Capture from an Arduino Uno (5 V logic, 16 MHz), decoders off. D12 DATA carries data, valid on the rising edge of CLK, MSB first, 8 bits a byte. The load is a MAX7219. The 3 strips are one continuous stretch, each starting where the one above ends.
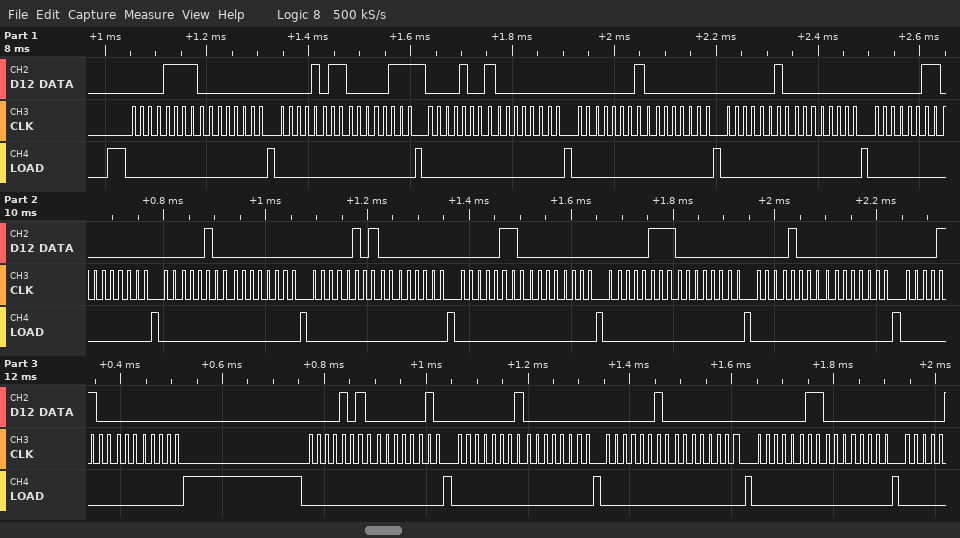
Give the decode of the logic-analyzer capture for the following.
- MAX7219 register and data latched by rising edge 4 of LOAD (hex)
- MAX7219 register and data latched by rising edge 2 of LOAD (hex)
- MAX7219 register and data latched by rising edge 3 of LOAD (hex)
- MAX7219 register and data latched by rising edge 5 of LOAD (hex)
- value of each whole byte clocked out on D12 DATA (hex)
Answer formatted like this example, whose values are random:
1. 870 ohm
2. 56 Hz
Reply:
1. register 0x9, data 0x00
2. register 0xF, data 0x00
3. register 0xB, data 0x07
4. register 0x1, data 0x00
5. 0x0F 0x00 0x0B 0x07 0x09 0x00 0x01 0x00 0x02 0x00 0x03 0x00 0x04 0x00 0x05 0x00 0x06 0x00 0x07 0x00 0x08 0x00 0x0C 0x00 0x0A 0x02 0x01 0x00 0x02 0x00 0x03 0x00
